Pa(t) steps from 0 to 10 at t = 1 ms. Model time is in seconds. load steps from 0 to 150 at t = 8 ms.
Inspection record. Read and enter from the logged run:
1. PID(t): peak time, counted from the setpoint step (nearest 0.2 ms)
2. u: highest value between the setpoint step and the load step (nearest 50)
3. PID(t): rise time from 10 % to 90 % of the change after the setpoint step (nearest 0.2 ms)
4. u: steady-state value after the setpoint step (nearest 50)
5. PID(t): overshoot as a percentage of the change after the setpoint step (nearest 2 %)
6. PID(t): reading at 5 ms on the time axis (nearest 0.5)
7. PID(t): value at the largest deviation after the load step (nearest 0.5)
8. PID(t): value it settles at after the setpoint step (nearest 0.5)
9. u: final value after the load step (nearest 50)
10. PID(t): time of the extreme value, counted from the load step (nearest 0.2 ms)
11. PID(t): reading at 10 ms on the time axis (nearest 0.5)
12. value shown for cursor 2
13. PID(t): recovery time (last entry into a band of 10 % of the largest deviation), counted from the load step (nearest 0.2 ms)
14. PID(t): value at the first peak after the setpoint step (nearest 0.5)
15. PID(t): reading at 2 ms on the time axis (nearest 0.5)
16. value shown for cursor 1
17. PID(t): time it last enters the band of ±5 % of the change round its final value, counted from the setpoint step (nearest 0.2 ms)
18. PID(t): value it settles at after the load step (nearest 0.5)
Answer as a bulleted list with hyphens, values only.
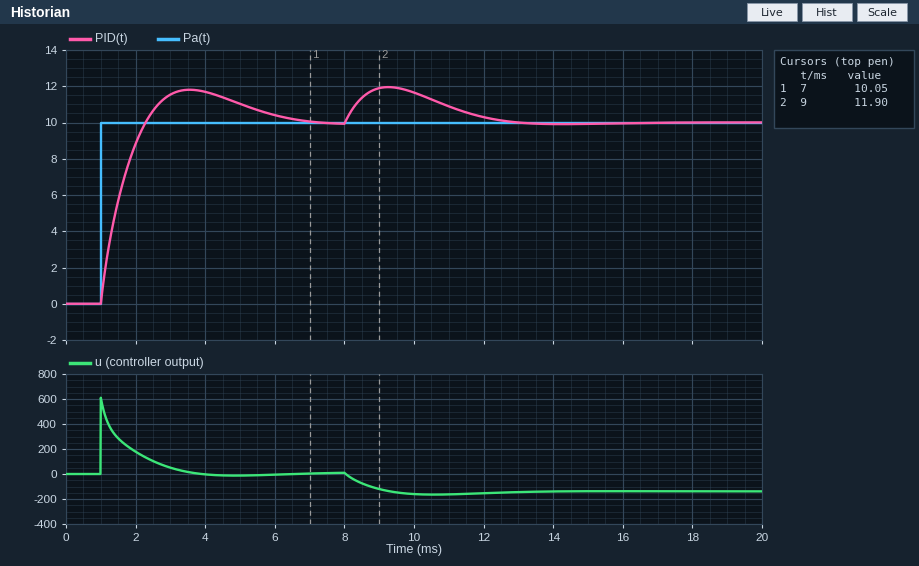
- 2.6 ms
- 600
- 1.0 ms
- 0
- 18 %
- 11.0
- 12.0
- 10.0
- -150
- 1.2 ms
- 11.5
- 11.90
- 4.2 ms
- 12.0
- 9.0
- 10.05
- 4.8 ms
- 10.0
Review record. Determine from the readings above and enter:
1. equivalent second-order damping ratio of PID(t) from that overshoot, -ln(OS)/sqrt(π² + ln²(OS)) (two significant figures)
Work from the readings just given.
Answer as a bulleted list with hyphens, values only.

- 0.48
